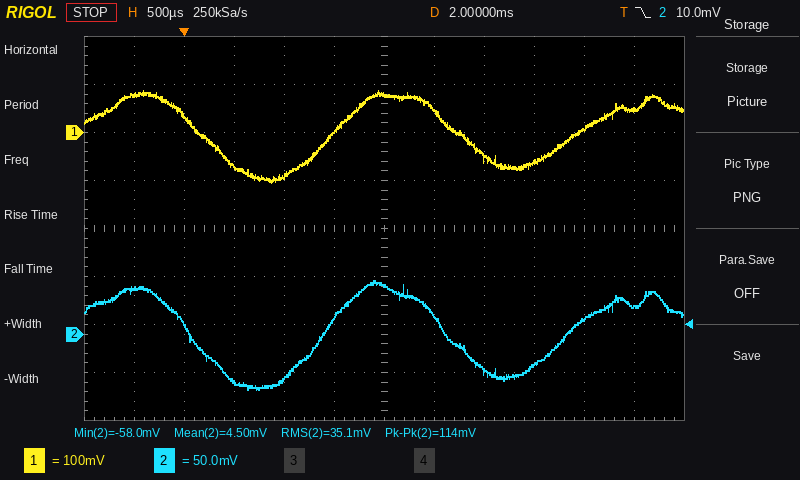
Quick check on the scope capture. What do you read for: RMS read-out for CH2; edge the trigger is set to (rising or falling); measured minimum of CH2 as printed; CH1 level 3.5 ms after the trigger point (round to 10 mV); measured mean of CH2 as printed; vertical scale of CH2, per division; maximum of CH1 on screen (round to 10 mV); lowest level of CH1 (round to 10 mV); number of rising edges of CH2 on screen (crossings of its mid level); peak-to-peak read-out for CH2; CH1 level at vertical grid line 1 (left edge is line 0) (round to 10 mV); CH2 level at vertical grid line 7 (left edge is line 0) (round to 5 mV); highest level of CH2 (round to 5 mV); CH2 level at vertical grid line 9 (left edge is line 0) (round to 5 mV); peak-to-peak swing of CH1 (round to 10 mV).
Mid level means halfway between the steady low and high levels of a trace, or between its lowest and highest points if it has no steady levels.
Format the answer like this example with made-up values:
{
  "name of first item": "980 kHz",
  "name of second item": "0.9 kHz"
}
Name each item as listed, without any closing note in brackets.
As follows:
{
  "RMS read-out for CH2": "35.1 mV",
  "edge the trigger is set to": "falling",
  "measured minimum of CH2 as printed": "-58.0 mV",
  "CH1 level 3.5 ms after the trigger point": "-60 mV",
  "measured mean of CH2 as printed": "4.50 mV",
  "vertical scale of CH2, per division": "50 mV",
  "maximum of CH1 on screen": "90 mV",
  "lowest level of CH1": "-100 mV",
  "number of rising edges of CH2 on screen": "2",
  "peak-to-peak read-out for CH2": "114 mV",
  "CH1 level at vertical grid line 1 (left edge is line 0)": "80 mV",
  "CH2 level at vertical grid line 7 (left edge is line 0)": "20 mV",
  "highest level of CH2": "55 mV",
  "CH2 level at vertical grid line 9 (left edge is line 0)": "-30 mV",
  "peak-to-peak swing of CH1": "190 mV"
}
